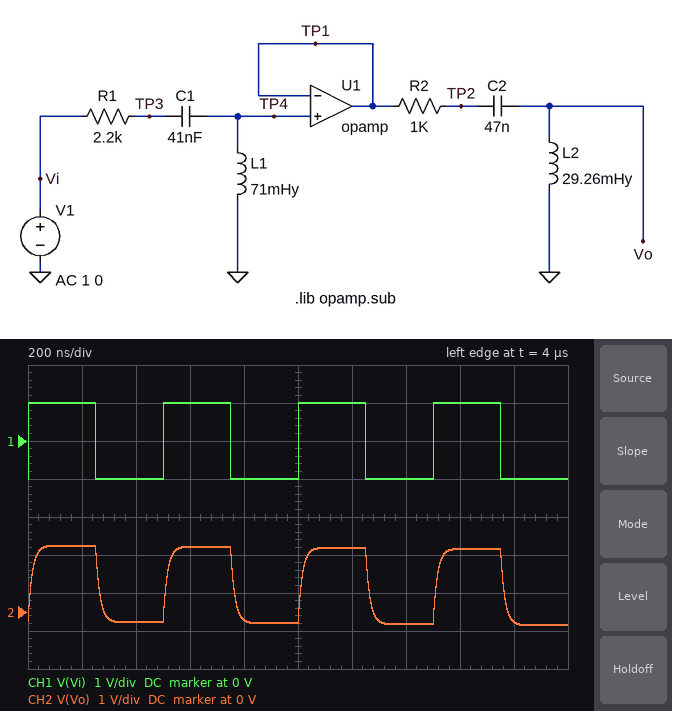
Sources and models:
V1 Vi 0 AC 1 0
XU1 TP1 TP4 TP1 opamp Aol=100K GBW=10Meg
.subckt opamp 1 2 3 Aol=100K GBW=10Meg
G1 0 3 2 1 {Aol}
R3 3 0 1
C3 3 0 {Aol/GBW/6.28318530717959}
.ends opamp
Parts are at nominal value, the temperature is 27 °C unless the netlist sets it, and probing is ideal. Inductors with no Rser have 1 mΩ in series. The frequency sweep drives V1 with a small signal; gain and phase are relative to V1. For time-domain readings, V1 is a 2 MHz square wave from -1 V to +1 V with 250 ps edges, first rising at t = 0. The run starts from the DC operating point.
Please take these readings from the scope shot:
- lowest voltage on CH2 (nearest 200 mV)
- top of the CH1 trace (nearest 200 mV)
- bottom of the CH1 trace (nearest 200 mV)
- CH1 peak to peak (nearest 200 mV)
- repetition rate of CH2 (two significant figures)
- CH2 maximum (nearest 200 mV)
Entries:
-400 mV
1.0 V
-1.0 V
2.0 V
2.0 MHz
1.8 V
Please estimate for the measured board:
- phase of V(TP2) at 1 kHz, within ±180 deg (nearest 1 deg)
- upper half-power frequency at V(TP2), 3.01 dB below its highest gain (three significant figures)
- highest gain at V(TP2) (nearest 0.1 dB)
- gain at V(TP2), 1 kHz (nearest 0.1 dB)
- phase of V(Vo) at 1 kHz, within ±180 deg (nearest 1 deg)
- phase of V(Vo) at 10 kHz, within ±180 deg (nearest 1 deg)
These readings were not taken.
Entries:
130 deg
10.0 MHz
0 dB
-19.6 dB
-50 deg
62 deg
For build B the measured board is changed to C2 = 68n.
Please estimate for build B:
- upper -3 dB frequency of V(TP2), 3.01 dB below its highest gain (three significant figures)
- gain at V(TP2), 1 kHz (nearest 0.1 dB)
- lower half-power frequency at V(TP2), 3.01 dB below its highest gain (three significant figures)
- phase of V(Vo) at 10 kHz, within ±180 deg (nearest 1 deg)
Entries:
10.0 MHz
-20.1 dB
7.83 kHz
60 deg
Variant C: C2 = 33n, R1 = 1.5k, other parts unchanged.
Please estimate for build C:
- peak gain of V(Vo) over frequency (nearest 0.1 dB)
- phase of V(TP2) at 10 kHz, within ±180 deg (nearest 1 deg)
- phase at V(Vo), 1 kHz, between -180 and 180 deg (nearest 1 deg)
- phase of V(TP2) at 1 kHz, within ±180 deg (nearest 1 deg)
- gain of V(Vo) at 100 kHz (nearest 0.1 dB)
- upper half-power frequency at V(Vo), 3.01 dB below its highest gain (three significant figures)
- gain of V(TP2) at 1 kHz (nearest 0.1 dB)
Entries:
1.3 dB
57 deg
-36 deg
144 deg
0 dB
6.95 MHz
-18.7 dB
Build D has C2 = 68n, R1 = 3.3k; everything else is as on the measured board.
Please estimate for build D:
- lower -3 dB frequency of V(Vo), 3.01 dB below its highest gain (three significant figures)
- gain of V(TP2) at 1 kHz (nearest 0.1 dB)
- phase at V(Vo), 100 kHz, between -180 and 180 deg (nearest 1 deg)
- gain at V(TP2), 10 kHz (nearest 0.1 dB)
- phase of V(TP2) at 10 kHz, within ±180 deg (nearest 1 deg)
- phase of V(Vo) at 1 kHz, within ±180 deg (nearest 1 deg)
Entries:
7.17 kHz
-21.4 dB
7 deg
-2.8 dB
71 deg
-69 deg
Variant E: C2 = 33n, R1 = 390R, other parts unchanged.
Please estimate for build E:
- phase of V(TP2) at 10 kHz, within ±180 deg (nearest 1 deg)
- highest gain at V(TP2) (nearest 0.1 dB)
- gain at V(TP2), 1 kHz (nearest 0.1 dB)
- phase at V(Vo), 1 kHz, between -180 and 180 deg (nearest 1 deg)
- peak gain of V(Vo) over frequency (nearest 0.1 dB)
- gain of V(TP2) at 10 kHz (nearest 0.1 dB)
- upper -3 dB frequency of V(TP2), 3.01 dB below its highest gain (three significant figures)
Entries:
42 deg
7.9 dB
-18.0 dB
-19 deg
2.9 dB
-1.1 dB
3.39 kHz
